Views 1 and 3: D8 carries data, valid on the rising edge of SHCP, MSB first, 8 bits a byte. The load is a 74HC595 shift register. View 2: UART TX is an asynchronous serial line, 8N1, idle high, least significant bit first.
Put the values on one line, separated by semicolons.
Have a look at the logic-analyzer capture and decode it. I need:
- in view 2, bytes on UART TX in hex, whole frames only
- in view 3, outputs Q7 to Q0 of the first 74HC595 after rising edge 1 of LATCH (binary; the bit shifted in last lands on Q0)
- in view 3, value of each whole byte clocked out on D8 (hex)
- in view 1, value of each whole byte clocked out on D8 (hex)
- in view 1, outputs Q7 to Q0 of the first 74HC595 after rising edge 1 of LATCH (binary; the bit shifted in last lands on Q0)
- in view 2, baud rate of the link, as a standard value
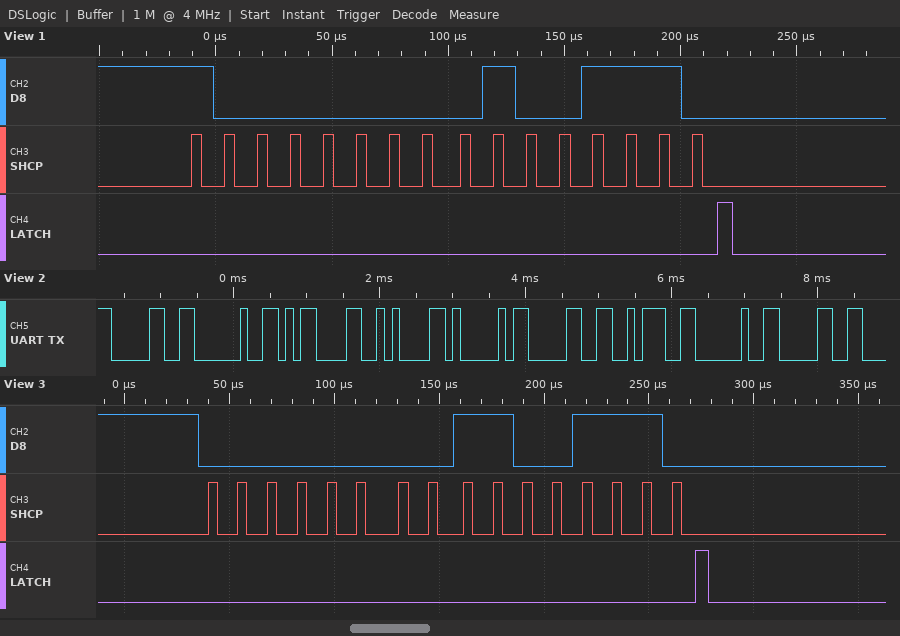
0x30 0x20 0x0D 0x0A 0x41 0x30 0x3A 0x20 0x30; 11001110; 00 CE; 80 4E; 01001110; 9600 baud
